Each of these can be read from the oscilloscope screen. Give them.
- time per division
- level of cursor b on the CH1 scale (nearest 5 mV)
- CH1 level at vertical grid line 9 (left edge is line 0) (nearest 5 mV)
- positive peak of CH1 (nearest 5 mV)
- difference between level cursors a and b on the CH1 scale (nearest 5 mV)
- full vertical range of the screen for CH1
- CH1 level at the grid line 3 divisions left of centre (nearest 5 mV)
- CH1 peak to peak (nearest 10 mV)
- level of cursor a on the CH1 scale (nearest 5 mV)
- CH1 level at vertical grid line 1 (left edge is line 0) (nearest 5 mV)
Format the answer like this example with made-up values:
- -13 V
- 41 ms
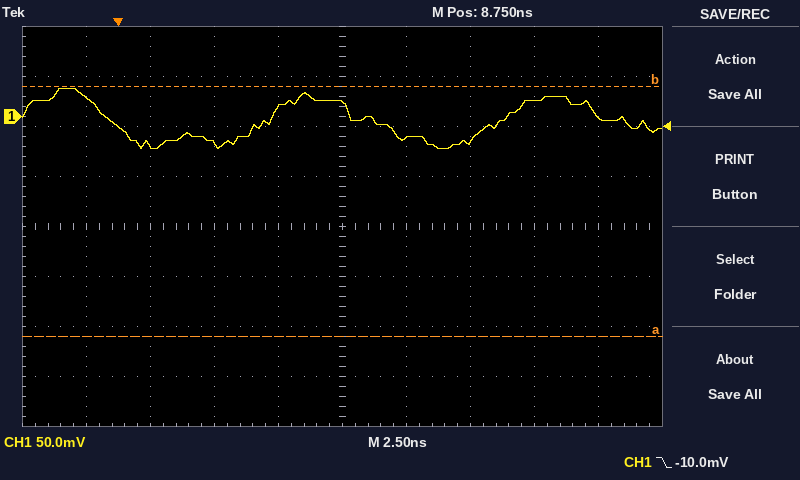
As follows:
- 2.5 ns
- 30 mV
- 0 mV
- 30 mV
- 250 mV
- 400 mV
- -30 mV
- 60 mV
- -220 mV
- 20 mV
